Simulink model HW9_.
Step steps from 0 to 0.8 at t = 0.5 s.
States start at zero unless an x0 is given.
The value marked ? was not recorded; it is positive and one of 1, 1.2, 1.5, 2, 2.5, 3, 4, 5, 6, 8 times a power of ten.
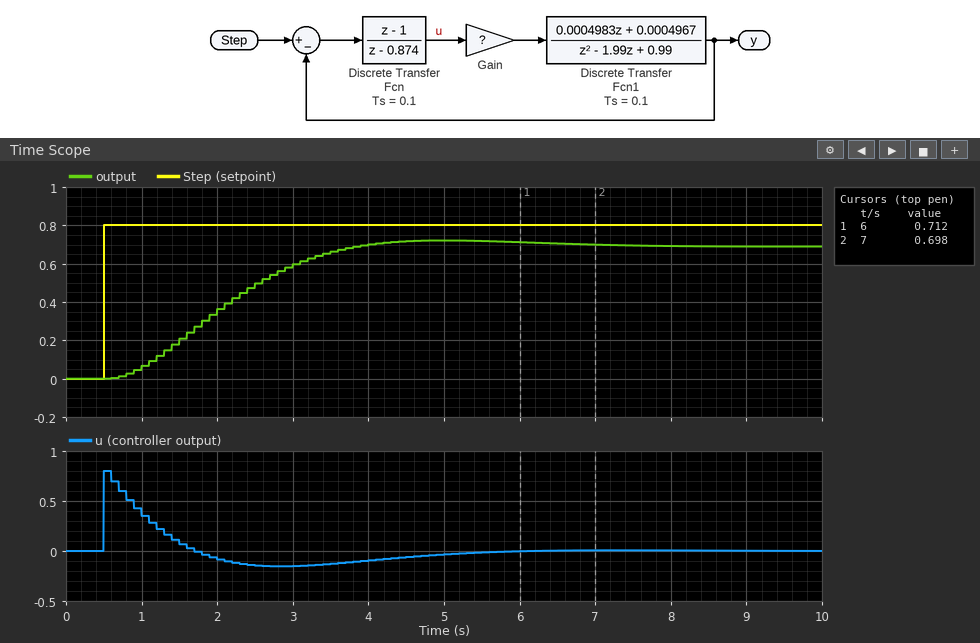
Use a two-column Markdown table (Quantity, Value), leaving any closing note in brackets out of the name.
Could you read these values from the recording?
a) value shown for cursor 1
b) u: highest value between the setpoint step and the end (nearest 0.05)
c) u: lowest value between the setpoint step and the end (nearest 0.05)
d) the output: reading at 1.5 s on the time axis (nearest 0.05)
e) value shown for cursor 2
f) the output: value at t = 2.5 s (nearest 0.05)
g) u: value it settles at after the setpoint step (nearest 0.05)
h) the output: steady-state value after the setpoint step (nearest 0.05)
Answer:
| Quantity | Value |
|---|---|
| value shown for cursor 1 | 0.712 |
| u: highest value between the setpoint step and the end | 0.80 |
| u: lowest value between the setpoint step and the end | -0.15 |
| the output: reading at 1.5 s on the time axis | 0.20 |
| value shown for cursor 2 | 0.698 |
| the output: value at t = 2.5 s | 0.50 |
| u: value it settles at after the setpoint step | 0.00 |
| the output: steady-state value after the setpoint step | 0.70 |
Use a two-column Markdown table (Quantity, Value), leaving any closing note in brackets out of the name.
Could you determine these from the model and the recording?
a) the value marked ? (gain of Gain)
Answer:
| Quantity | Value |
|---|---|
| the value marked ? | 8 |
